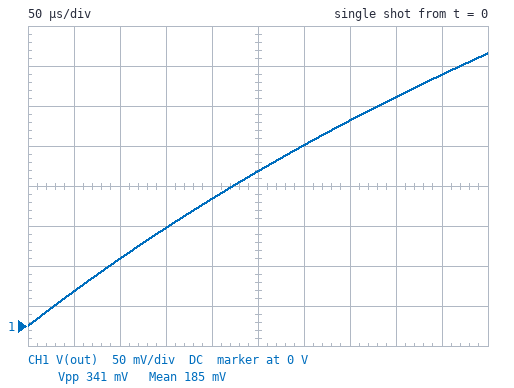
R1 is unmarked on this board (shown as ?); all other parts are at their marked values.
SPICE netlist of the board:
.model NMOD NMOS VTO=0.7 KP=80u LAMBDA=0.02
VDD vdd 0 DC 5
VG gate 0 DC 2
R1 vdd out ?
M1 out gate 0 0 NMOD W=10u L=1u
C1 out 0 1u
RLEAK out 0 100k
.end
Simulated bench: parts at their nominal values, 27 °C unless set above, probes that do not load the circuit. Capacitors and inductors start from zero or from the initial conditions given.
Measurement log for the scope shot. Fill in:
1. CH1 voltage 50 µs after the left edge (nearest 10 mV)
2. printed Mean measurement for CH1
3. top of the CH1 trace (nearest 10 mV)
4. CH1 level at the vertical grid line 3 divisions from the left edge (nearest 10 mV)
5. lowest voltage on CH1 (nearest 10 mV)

40 mV
185 mV
340 mV
120 mV
0 V
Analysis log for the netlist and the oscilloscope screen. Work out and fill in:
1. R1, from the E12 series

5.6 kΩ
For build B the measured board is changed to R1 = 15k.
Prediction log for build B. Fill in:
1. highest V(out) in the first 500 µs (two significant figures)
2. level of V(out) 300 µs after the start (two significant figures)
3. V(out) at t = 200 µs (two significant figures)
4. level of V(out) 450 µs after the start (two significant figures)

130 mV
85 mV
60 mV
120 mV
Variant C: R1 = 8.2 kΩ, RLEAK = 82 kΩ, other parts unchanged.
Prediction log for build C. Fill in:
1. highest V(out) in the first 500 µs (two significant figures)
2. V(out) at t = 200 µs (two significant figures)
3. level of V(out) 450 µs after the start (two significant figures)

230 mV
110 mV
220 mV
